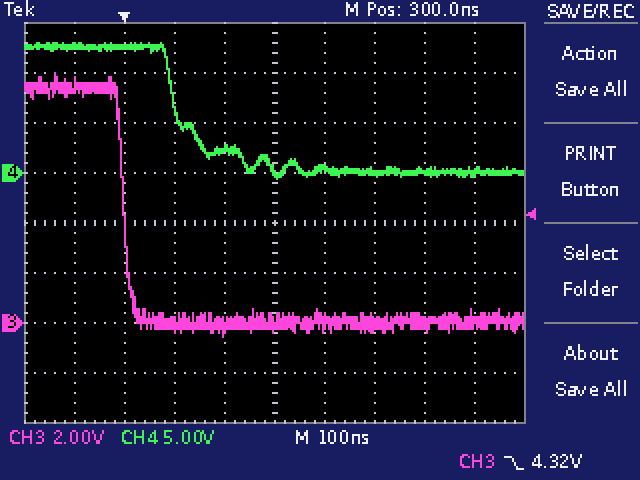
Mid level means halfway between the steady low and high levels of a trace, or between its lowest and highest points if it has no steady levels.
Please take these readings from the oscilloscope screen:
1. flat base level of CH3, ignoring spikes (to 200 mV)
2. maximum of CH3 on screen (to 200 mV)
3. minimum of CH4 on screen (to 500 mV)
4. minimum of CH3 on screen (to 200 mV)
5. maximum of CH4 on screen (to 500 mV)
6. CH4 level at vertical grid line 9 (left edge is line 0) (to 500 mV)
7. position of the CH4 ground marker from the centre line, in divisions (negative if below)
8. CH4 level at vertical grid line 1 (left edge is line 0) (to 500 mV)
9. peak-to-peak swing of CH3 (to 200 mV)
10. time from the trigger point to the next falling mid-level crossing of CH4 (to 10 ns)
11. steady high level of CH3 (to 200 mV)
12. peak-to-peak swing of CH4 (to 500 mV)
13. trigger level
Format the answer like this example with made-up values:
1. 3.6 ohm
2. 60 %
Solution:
1. 0.0 V
2. 10.0 V
3. -500 mV
4. -600 mV
5. 13.0 V
6. 0.0 V
7. +1.0 div
8. 12.5 V
9. 10.6 V
10. 100 ns
11. 9.4 V
12. 13.5 V
13. 4.32 V
